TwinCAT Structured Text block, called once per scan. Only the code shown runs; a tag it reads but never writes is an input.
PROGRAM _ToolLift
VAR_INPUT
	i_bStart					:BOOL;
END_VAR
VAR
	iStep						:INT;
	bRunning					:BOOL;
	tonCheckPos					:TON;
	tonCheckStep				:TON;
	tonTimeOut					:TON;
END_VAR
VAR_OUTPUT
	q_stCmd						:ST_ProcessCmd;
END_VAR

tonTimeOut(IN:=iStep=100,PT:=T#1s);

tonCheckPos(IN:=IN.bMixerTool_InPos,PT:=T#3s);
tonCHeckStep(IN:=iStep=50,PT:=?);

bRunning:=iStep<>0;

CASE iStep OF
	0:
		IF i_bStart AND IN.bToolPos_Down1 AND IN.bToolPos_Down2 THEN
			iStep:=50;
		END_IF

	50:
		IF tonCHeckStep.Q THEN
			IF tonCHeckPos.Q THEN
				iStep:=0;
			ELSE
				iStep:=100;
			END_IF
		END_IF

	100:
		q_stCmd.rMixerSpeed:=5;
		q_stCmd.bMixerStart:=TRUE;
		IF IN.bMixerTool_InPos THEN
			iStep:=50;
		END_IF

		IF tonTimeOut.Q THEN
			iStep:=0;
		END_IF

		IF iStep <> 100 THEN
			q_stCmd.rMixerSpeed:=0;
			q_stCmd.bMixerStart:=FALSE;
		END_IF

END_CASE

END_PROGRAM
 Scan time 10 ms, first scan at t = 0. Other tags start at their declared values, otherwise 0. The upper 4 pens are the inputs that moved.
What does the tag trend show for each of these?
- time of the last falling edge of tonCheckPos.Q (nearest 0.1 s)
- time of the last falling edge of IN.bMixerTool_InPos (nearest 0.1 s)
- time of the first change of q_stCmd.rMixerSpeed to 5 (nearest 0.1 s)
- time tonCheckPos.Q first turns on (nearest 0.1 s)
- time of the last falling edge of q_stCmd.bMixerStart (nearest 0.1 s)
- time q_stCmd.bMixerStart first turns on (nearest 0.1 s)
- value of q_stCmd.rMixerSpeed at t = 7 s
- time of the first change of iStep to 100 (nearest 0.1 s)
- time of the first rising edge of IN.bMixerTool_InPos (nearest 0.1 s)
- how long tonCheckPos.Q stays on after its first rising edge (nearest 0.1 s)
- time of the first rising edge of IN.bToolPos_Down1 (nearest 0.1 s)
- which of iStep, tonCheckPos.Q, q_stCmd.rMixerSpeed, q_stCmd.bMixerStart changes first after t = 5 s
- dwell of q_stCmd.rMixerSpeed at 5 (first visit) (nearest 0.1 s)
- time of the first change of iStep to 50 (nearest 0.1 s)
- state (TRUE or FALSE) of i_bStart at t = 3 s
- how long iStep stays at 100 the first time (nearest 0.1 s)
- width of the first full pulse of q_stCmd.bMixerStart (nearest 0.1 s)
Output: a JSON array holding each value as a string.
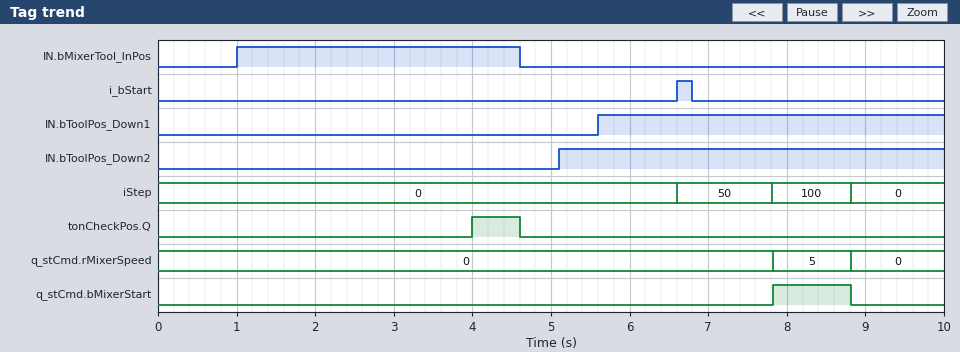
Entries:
["4.6 s", "4.6 s", "7.8 s", "4.0 s", "8.8 s", "7.8 s", "0", "7.8 s", "1.0 s", "0.6 s", "5.6 s", "iStep", "1.0 s", "6.6 s", "FALSE", "1.0 s", "1.0 s"]
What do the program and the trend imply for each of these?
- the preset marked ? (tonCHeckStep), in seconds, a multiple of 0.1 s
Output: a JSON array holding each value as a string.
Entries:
["1.2 s"]
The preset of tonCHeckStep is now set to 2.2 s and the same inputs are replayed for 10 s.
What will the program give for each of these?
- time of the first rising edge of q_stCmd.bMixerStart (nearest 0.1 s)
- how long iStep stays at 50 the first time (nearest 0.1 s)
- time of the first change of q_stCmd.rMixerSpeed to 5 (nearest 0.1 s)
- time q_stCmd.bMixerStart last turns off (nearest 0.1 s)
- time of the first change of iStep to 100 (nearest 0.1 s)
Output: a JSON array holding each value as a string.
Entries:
["8.8 s", "2.2 s", "8.8 s", "9.8 s", "8.8 s"]
